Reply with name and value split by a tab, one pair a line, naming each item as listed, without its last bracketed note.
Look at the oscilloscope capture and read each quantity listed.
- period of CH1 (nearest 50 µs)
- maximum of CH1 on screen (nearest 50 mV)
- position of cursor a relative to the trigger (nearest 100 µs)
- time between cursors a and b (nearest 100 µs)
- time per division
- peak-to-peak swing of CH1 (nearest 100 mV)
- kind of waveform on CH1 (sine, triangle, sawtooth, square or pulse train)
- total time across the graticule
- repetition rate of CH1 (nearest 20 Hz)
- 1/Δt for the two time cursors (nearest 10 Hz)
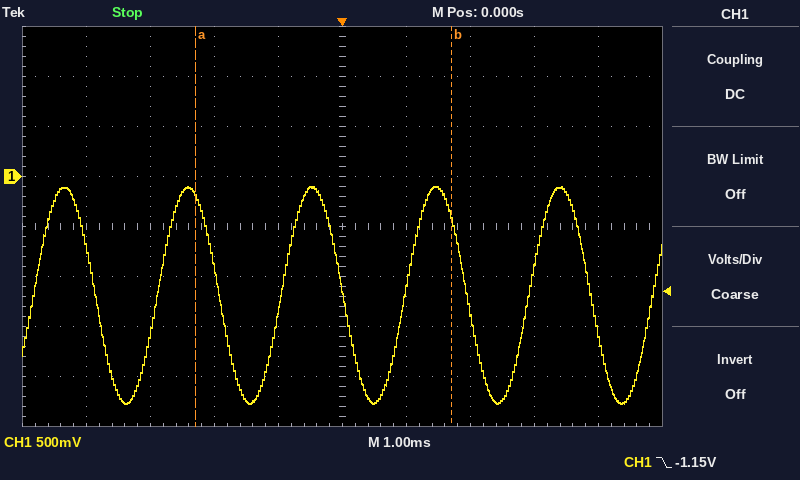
period of CH1	1.95 ms
maximum of CH1 on screen	-100 mV
position of cursor a relative to the trigger	-2.3 ms
time between cursors a and b	4.0 ms
time per division	1 ms
peak-to-peak swing of CH1	2.20 V
kind of waveform on CH1	sine
total time across the graticule	10 ms
repetition rate of CH1	520 Hz
1/Δt for the two time cursors	250 Hz
